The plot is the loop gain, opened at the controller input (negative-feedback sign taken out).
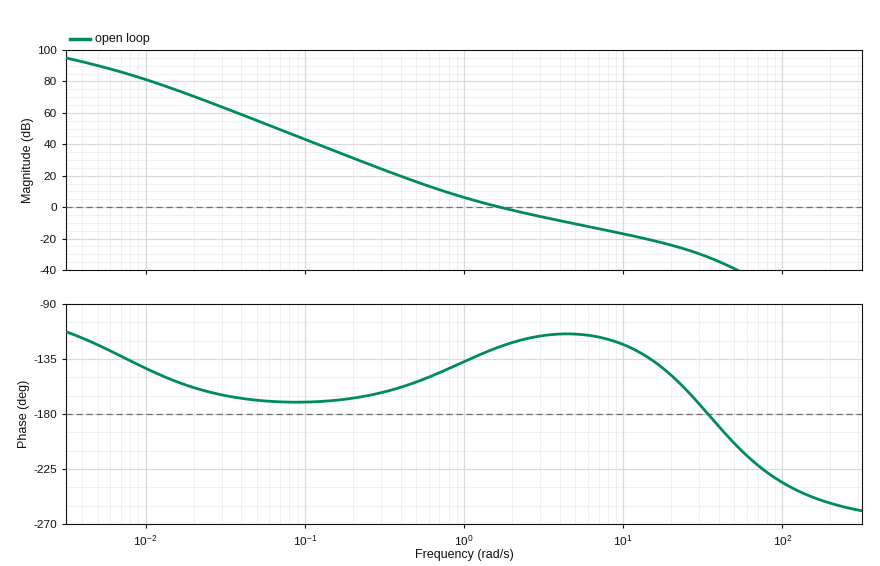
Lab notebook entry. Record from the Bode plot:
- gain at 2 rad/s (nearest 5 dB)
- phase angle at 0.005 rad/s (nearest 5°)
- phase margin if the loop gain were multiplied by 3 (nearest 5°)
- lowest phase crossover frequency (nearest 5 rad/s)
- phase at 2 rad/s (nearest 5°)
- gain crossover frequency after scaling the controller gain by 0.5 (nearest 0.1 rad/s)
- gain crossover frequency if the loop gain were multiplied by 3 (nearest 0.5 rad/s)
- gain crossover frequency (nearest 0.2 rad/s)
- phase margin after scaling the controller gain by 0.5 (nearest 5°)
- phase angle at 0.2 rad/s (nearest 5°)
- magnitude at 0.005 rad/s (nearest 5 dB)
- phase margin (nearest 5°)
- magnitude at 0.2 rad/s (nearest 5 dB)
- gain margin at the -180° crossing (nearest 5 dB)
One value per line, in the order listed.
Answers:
0 dB
-125°
65°
35 rad/s
-120°
1.0 rad/s
4.5 rad/s
1.6 rad/s
45°
-165°
90 dB
55°
30 dB
30 dB
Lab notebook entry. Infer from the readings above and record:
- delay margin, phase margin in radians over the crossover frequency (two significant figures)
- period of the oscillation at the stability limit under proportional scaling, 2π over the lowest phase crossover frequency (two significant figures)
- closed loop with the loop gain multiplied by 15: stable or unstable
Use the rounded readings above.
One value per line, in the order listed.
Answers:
0.60 s
0.18 s
stable
